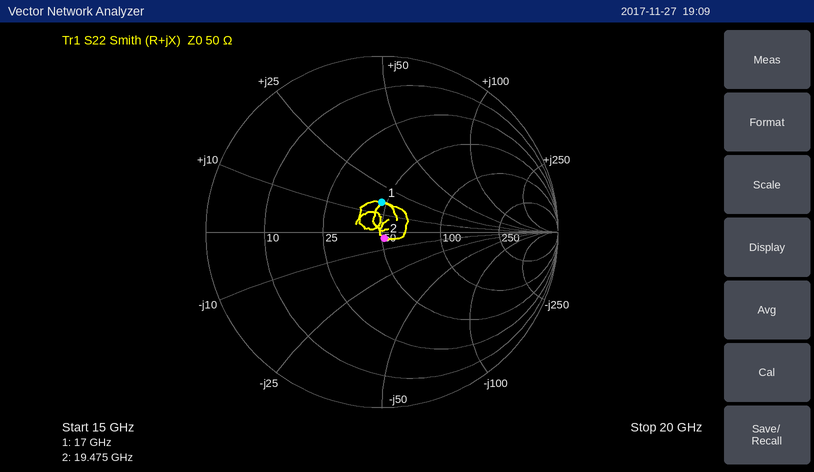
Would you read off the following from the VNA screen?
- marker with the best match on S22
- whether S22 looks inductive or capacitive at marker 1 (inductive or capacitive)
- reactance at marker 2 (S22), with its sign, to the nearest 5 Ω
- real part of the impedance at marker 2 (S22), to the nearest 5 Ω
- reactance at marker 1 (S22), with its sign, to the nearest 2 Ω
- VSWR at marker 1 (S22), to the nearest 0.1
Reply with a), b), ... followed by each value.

a) marker 2
b) inductive
c) -5 Ω
d) 50 Ω
e) +16 Ω
f) 1.4
